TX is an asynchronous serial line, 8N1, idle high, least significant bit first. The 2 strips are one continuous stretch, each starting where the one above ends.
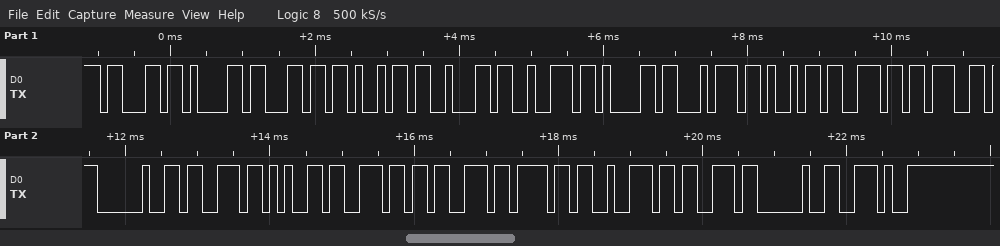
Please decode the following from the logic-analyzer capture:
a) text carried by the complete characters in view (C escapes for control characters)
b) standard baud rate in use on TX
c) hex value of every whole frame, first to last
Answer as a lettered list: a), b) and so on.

a) "calibrating sensors ."
b) 9600 baud
c) 0x63 0x61 0x6C 0x69 0x62 0x72 0x61 0x74 0x69 0x6E 0x67 0x20 0x73 0x65 0x6E 0x73 0x6F 0x72 0x73 0x20 0x2E
